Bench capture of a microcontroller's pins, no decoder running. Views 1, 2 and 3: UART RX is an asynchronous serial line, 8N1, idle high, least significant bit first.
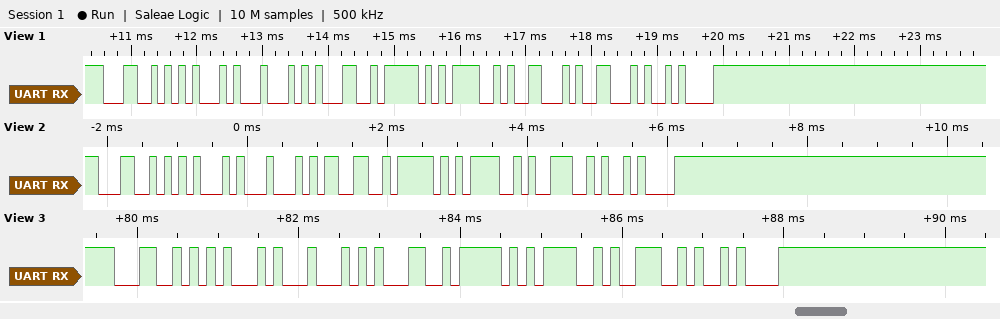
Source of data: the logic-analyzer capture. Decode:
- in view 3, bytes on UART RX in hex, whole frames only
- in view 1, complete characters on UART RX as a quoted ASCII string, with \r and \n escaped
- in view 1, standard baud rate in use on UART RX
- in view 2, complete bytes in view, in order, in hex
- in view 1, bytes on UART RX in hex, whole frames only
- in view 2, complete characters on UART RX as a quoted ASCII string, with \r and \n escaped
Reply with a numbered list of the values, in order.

1. 4C 45 44 31 5F 4F 4E 0A
2. "LED1_OFF\n"
3. 9600 baud
4. 4C 45 44 33 5F 4F 4E 0A
5. 4C 45 44 31 5F 4F 46 46 0A
6. "LED3_ON\n"
